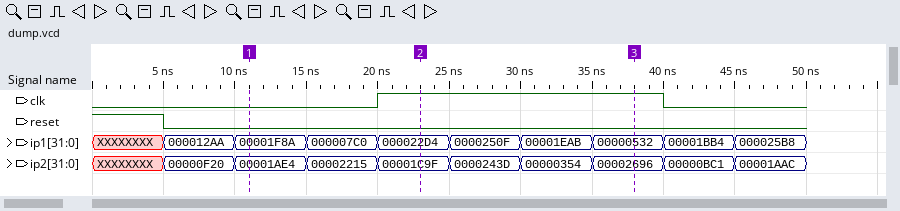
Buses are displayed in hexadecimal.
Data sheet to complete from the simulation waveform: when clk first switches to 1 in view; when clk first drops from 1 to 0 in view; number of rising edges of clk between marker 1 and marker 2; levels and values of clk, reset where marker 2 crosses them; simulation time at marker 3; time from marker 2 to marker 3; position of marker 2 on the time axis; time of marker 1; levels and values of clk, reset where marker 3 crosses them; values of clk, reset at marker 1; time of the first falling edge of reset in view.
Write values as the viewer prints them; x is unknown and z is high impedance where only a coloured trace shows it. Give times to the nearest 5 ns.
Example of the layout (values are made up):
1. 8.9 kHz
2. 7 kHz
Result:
1. 20 ns
2. 40 ns
3. 1
4. clk=1, reset=0
5. 40 ns
6. 15 ns
7. 25 ns
8. 10 ns
9. clk=1, reset=0
10. clk=0, reset=0
11. 5 ns
